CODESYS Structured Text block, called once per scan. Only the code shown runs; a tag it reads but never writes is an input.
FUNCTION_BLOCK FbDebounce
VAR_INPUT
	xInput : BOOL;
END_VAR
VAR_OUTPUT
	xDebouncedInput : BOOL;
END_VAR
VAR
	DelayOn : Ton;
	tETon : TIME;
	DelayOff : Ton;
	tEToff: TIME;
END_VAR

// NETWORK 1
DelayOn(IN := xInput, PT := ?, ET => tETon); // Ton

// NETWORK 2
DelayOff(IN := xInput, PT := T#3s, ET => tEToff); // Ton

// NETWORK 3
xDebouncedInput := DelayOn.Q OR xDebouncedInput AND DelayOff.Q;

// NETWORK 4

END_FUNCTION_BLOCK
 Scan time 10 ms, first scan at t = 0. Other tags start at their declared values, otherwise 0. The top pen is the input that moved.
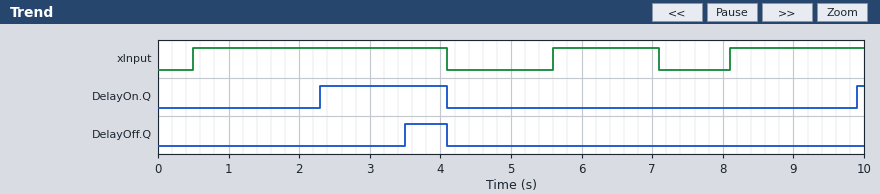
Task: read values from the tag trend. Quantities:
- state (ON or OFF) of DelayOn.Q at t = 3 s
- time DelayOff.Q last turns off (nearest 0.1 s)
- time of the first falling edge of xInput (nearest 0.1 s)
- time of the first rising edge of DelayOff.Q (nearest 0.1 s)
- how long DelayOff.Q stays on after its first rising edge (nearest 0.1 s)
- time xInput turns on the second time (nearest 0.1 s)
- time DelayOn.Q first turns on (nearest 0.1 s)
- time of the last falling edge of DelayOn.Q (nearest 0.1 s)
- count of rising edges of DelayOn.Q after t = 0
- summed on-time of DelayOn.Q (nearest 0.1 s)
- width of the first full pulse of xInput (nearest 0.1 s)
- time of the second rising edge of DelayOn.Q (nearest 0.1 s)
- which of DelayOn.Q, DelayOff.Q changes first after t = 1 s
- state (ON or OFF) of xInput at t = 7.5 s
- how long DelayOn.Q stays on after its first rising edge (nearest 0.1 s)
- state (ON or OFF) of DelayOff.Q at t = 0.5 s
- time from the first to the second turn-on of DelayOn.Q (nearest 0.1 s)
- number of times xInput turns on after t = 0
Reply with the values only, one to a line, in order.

ON
4.1 s
4.1 s
3.5 s
0.6 s
5.6 s
2.3 s
4.1 s
2
1.9 s
3.6 s
9.9 s
DelayOn.Q
OFF
1.8 s
OFF
7.6 s
3
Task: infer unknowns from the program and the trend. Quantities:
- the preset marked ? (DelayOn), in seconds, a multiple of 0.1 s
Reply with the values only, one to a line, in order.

1.8 s
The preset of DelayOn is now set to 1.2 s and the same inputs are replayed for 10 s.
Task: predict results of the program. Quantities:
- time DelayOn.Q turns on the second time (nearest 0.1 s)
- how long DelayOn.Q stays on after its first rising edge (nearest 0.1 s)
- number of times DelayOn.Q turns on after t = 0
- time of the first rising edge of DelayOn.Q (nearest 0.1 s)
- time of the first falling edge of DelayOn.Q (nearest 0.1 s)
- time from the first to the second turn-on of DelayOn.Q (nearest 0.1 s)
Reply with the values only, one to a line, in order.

6.8 s
2.4 s
3
1.7 s
4.1 s
5.1 s
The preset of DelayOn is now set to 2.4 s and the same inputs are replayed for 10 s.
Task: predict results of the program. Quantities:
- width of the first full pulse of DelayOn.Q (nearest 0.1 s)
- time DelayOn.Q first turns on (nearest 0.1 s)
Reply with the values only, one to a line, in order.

1.2 s
2.9 s
